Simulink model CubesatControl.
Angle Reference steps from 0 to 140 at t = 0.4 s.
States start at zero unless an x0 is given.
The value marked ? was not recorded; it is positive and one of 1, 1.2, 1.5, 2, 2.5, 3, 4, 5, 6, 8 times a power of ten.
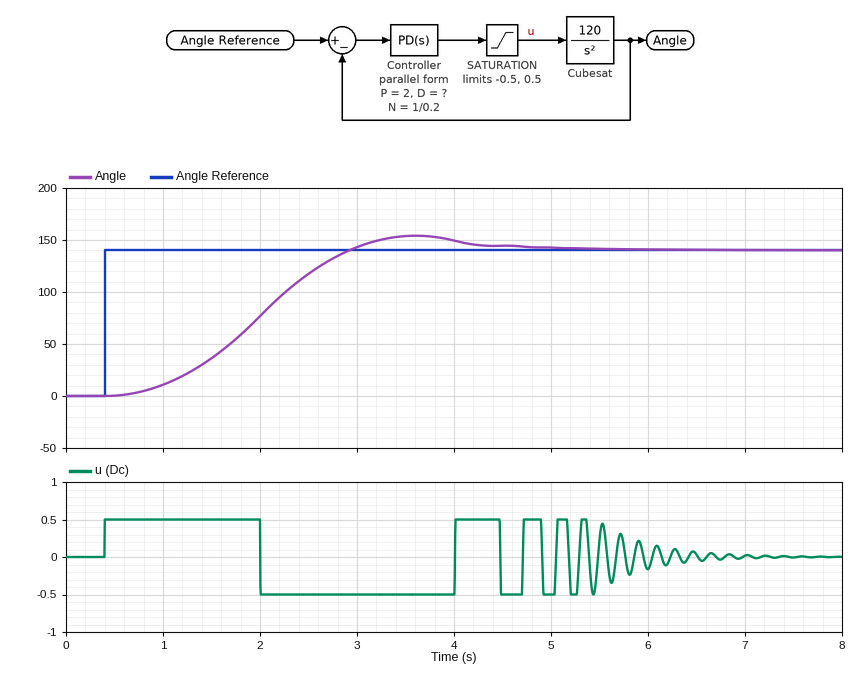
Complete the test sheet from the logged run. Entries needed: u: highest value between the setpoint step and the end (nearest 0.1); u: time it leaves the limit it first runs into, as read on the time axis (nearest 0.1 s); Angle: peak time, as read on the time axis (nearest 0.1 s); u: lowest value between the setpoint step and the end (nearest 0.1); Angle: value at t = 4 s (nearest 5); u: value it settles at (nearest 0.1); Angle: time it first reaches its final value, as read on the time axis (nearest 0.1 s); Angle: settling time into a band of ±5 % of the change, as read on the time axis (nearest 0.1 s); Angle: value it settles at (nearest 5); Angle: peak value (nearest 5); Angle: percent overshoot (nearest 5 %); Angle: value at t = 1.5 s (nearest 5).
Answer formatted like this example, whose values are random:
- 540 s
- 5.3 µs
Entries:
- 0.5
- 2.0 s
- 3.6 s
- -0.5
- 150
- 0.0
- 2.9 s
- 4.1 s
- 140
- 155
- 10 %
- 35
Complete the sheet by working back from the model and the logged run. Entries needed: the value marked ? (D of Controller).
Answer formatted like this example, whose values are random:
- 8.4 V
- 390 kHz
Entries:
- 1.5
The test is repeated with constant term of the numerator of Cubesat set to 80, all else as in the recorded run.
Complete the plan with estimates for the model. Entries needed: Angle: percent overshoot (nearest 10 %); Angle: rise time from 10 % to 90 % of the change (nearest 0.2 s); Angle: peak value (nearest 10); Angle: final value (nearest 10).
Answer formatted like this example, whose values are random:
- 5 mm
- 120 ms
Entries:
- 20 %
- 1.8 s
- 170
- 140
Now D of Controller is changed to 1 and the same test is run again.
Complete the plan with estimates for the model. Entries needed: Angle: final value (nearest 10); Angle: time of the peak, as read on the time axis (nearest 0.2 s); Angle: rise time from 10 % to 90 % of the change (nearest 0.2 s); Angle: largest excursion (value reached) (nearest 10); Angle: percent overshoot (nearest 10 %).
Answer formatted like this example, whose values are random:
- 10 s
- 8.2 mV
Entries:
- 140
- 4.0 s
- 1.4 s
- 190
- 30 %
